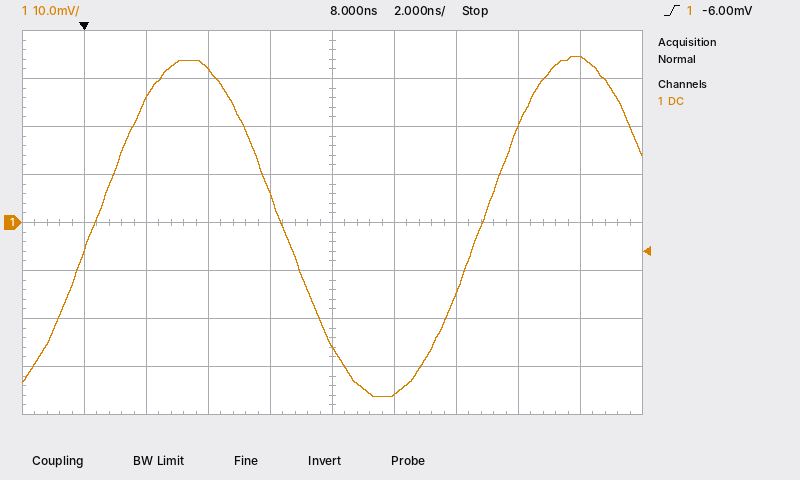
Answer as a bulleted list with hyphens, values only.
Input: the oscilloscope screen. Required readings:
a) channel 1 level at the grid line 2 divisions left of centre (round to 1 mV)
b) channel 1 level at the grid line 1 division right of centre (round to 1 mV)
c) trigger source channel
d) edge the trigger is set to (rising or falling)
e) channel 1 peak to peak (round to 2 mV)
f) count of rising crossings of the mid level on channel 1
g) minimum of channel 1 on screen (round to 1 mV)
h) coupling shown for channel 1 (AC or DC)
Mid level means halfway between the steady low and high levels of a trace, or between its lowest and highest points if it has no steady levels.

- 32 mV
- -36 mV
- channel 1
- rising
- 70 mV
- 2
- -36 mV
- DC
